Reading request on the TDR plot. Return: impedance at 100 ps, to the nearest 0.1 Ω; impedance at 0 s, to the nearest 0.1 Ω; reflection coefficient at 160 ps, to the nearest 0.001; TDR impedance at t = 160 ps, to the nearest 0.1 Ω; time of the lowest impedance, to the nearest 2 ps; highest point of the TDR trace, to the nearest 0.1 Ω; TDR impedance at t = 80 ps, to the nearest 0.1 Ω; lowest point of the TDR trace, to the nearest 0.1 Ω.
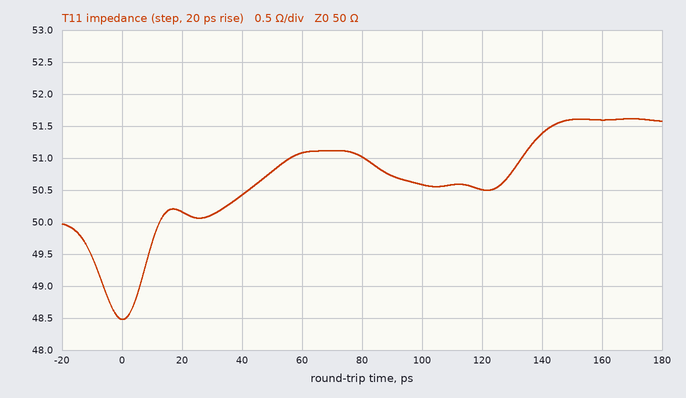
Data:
50.6 Ω
48.5 Ω
+0.016
51.6 Ω
0 ps
51.6 Ω
51.0 Ω
48.5 Ω
